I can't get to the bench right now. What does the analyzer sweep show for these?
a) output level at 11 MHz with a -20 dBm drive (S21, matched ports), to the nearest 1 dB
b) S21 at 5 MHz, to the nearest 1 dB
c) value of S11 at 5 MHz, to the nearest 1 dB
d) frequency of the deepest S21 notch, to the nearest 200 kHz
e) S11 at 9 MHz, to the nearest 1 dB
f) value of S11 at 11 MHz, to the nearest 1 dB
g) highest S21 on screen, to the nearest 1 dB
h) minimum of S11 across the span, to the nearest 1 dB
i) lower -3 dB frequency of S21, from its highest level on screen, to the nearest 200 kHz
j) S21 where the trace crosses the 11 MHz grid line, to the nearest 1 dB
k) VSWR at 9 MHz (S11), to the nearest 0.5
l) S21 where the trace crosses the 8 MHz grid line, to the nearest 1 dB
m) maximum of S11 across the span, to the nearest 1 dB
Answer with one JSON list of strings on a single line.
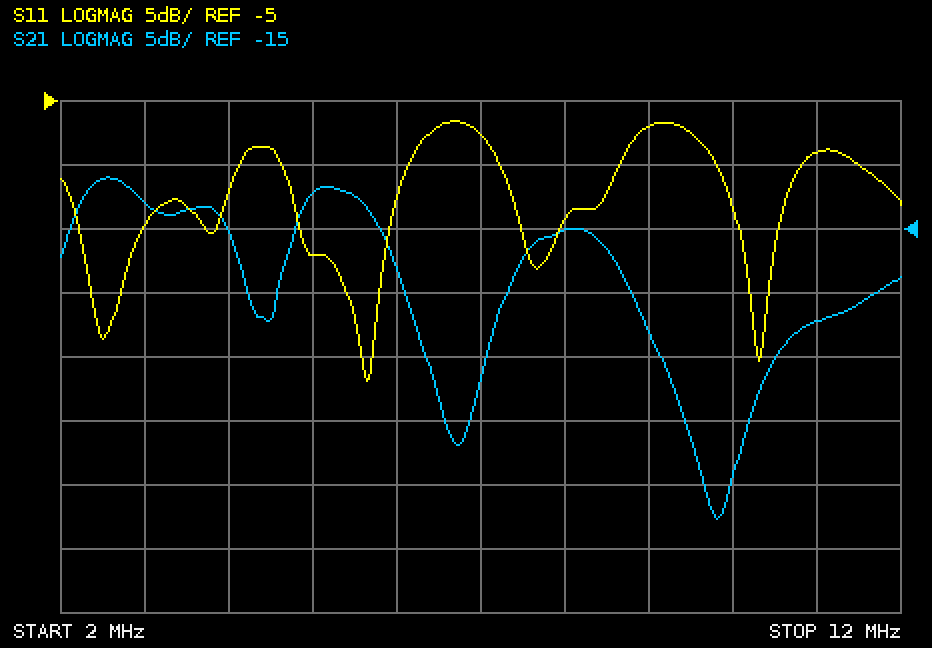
["-42 dBm", "-12 dB", "-17 dB", "9.8 MHz", "-7 dB", "-9 dB", "-11 dB", "-27 dB", "2.2 MHz", "-22 dB", "2.5", "-15 dB", "-7 dB"]
